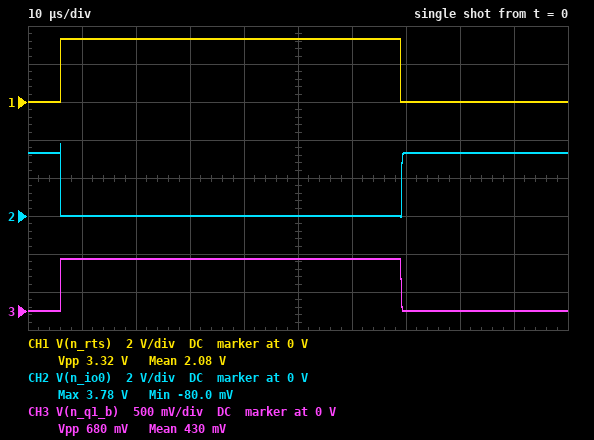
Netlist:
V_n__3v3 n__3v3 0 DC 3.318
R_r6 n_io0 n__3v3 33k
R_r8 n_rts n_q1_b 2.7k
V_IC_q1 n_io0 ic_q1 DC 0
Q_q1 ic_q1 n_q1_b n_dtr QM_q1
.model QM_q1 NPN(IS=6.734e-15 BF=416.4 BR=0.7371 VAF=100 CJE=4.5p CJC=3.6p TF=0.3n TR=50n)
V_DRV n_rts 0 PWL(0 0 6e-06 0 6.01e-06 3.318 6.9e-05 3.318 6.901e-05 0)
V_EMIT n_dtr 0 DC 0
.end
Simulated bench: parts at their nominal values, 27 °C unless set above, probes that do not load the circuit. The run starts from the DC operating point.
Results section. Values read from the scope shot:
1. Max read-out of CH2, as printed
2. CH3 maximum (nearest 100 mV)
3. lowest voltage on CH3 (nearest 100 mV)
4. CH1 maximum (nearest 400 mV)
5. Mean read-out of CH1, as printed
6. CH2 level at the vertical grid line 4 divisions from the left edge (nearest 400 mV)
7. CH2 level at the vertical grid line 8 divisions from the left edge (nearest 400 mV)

3.78 V
700 mV
0 V
3.2 V
2.08 V
0 V
3.2 V
